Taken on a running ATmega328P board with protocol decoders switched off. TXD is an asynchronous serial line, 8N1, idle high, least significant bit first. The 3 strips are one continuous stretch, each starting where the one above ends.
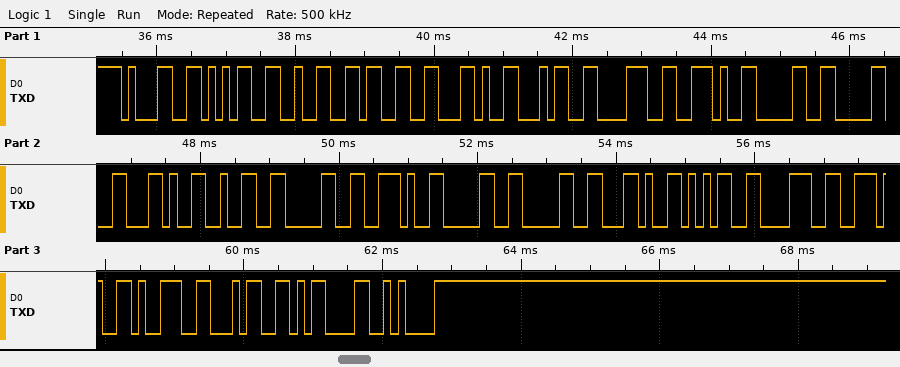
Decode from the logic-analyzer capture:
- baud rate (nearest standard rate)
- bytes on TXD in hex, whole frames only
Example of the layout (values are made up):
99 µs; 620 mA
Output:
9600 baud; 0x31 0x35 0x32 0x33 0x2C 0x34 0x38 0x2E 0x30 0x30 0x2C 0x32 0x30 0x2E 0x30 0x30 0x2C 0x35 0x38 0x2E 0x39 0x34 0x0D 0x0A
